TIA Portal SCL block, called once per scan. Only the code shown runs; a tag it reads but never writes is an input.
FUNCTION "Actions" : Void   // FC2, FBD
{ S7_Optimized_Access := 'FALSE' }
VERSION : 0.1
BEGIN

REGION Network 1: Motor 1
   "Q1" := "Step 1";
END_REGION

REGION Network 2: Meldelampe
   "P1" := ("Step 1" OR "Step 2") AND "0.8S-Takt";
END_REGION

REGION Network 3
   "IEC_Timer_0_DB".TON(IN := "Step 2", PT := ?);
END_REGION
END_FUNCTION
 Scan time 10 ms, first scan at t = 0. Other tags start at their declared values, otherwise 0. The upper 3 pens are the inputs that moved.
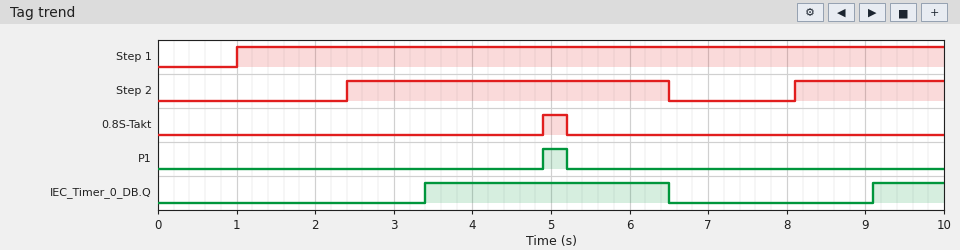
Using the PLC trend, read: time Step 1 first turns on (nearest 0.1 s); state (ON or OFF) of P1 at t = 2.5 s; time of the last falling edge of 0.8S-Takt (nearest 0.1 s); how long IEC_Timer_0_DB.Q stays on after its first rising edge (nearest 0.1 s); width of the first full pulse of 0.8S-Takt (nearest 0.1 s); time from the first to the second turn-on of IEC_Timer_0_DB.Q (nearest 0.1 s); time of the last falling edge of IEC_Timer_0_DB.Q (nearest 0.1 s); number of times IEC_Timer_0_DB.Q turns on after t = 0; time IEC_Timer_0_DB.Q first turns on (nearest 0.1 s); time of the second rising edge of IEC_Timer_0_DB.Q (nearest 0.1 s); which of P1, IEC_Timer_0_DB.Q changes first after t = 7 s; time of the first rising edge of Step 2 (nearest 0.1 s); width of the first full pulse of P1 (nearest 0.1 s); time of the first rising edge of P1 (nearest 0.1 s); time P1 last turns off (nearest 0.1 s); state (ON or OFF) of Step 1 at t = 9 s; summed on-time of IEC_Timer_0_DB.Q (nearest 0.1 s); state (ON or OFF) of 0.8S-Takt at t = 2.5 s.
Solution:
1.0 s
OFF
5.2 s
3.1 s
0.3 s
5.7 s
6.5 s
2
3.4 s
9.1 s
IEC_Timer_0_DB.Q
2.4 s
0.3 s
4.9 s
5.2 s
ON
4.0 s
OFF
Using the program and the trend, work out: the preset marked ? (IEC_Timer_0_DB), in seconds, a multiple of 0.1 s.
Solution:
1.0 s
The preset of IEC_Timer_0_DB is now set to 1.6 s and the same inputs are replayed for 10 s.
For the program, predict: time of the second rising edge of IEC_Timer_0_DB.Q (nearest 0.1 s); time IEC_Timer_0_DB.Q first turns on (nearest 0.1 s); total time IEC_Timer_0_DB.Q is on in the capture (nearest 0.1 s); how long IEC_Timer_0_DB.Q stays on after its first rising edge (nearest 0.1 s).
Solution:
9.7 s
4.0 s
2.8 s
2.5 s
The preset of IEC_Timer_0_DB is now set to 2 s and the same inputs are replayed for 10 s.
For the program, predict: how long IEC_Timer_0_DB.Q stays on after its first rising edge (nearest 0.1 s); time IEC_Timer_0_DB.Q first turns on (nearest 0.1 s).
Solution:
2.1 s
4.4 s
